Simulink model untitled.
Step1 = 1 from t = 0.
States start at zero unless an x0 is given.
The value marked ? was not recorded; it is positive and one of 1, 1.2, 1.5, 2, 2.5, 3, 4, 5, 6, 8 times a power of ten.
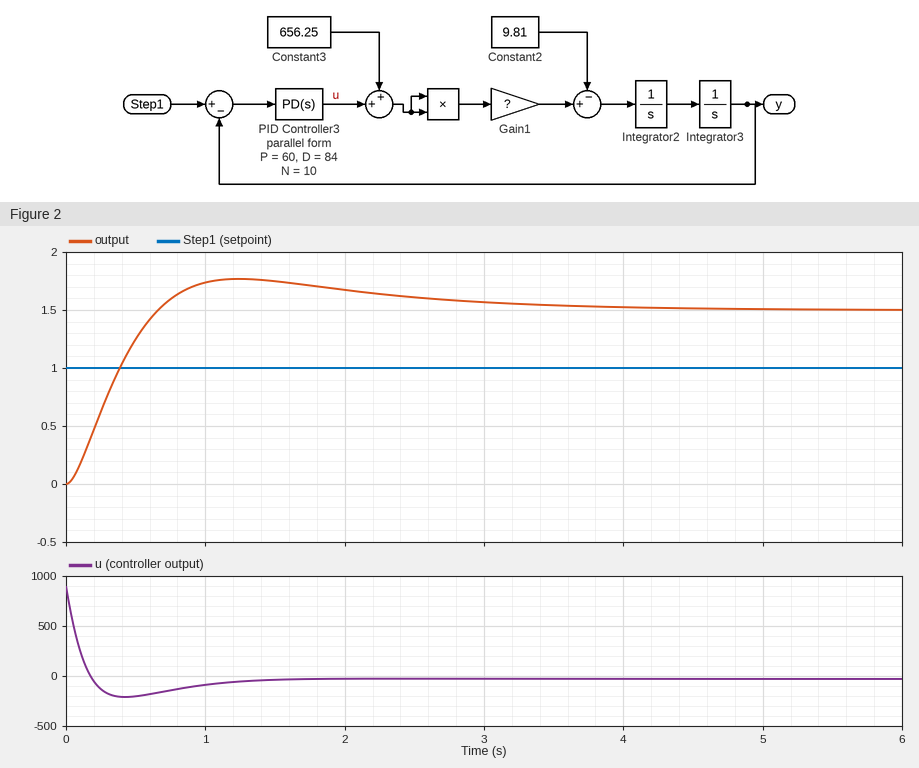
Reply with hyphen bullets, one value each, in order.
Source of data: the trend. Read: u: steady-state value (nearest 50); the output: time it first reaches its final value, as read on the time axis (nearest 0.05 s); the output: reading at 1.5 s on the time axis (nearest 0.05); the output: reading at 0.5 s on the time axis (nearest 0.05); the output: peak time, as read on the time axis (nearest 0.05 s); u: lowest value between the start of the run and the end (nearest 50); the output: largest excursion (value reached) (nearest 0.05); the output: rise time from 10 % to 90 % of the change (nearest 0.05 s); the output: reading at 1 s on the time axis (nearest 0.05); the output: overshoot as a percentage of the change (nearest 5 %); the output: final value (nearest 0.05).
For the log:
- -50
- 0.65 s
- 1.75
- 1.25
- 1.25 s
- -200
- 1.75
- 0.45 s
- 1.75
- 20 %
- 1.50
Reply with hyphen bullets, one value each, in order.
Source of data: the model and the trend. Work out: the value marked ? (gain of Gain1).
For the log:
- 2.5e-05
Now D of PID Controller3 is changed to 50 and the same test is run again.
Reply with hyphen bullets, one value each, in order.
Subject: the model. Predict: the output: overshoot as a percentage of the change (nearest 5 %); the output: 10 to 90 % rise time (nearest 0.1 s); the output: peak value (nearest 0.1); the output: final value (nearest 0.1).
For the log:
- 25 %
- 0.6 s
- 1.9
- 1.5
